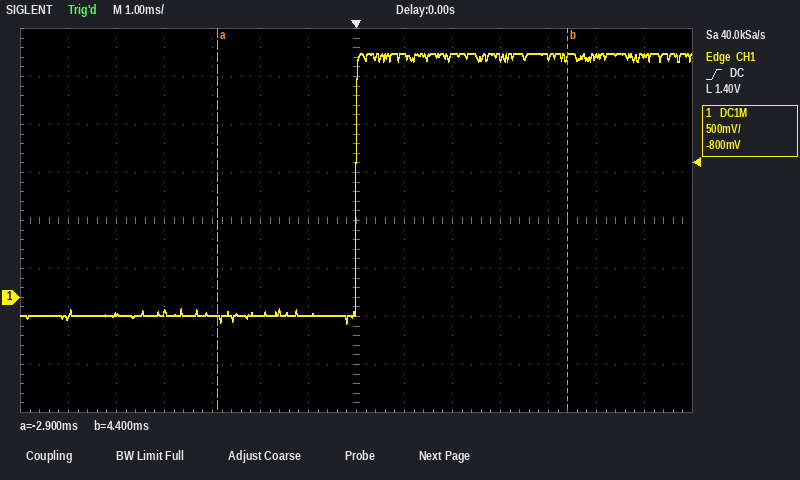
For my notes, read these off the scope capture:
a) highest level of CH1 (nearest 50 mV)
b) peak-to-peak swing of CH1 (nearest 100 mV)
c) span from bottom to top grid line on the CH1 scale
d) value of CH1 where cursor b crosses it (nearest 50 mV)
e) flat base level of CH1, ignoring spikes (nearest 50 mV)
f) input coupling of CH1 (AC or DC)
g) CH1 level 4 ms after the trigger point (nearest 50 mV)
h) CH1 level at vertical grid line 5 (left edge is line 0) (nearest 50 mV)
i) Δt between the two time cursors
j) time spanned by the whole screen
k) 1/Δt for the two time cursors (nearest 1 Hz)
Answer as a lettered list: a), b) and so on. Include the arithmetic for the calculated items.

a) 2.55 V
b) 2.80 V
c) 4 V
d) 2.50 V
e) -200 mV
f) DC
g) 2.50 V
h) -200 mV
i) 4.4 ms − (-2.9 ms) = 7.3 ms
j) 14 ms
k) 1 / 7.3 ms ≈ 137 Hz
